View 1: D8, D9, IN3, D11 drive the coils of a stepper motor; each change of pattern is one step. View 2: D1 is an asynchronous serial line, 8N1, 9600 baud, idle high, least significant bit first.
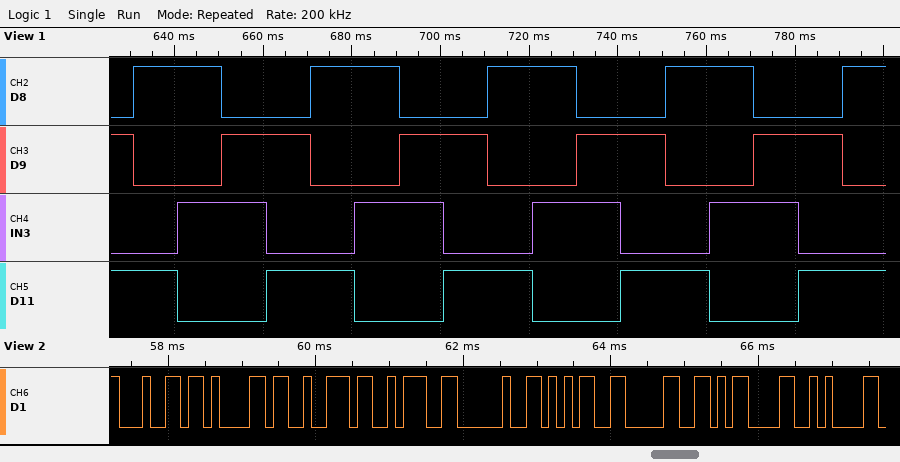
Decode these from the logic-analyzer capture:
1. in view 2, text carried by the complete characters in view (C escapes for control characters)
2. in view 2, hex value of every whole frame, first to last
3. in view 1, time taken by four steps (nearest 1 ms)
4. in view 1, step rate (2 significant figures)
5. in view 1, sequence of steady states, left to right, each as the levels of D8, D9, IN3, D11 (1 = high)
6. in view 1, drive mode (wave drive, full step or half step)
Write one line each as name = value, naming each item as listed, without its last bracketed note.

in view 2, text carried by the complete characters in view = "dar: 50\r\n"
in view 2, hex value of every whole frame, first to last = 0x64 0x61 0x72 0x3A 0x20 0x35 0x30 0x0D 0x0A
in view 1, time taken by four steps = 40 ms
in view 1, step rate = 100 steps/s
in view 1, sequence of steady states, left to right, each as the levels of D8, D9, IN3, D11 = 0101 1001 1010 0110 0101 1001 1010 0110 0101 1001 1010 0110 0101 1001 1010 0110 0101 1001
in view 1, drive mode = full step
